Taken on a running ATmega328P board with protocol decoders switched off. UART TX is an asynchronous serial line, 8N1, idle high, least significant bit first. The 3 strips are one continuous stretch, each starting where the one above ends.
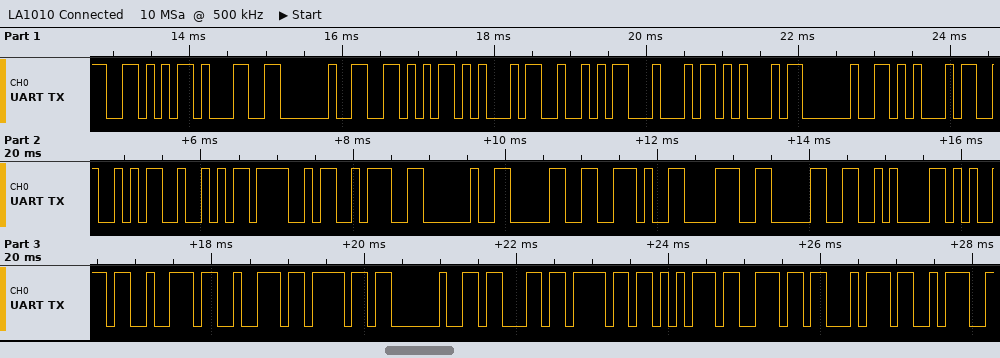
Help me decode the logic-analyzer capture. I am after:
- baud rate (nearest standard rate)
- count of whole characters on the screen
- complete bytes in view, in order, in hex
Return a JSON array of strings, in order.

["9600 baud", "31", "56 31 20 56 45 52 44 45 20 45 52 52 4F 3A 20 30 2E 38 30 0A 65 72 72 6F 20 63 6F 75 6E 74 3A"]
